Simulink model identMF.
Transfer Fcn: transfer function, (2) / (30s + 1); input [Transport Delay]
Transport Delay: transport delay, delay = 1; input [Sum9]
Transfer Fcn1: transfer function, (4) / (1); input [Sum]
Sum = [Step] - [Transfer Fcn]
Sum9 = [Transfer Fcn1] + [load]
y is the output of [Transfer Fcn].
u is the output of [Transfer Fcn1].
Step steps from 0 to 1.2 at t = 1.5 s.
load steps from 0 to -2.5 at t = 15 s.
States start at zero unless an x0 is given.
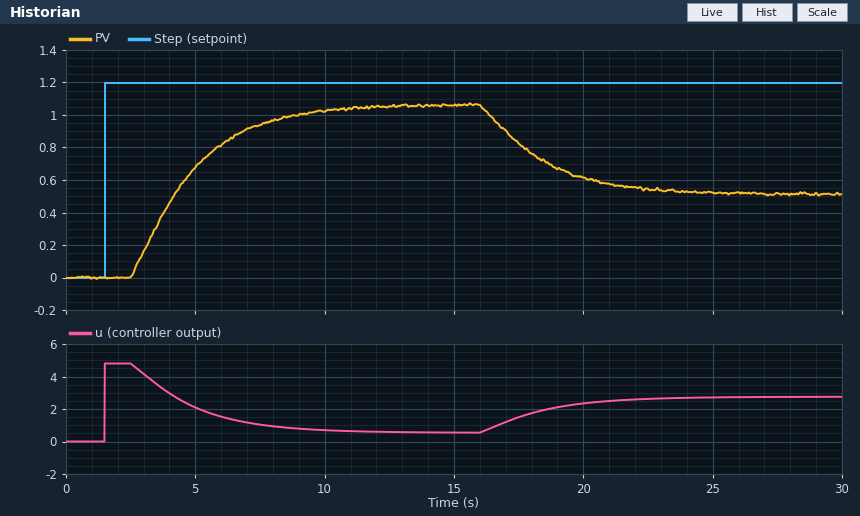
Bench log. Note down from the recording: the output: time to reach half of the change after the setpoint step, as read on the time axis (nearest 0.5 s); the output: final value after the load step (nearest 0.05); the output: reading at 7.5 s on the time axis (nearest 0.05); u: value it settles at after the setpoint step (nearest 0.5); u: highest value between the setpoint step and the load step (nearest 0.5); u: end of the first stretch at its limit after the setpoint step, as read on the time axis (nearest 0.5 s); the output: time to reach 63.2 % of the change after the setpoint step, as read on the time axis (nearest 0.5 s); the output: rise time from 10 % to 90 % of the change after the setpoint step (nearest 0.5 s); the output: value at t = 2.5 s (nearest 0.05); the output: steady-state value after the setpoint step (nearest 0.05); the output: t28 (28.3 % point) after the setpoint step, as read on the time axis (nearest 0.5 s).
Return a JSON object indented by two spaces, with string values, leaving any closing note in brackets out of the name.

{
  "the output: time to reach half of the change after the setpoint step, as read on the time axis": "4.5 s",
  "the output: final value after the load step": "0.50",
  "the output: reading at 7.5 s on the time axis": "0.95",
  "u: value it settles at after the setpoint step": "0.5",
  "u: highest value between the setpoint step and the load step": "5.0",
  "u: end of the first stretch at its limit after the setpoint step, as read on the time axis": "2.5 s",
  "the output: time to reach 63.2 % of the change after the setpoint step, as read on the time axis": "5.0 s",
  "the output: rise time from 10 % to 90 % of the change after the setpoint step": "5.0 s",
  "the output: value at t = 2.5 s": "0.00",
  "the output: steady-state value after the setpoint step": "1.05",
  "the output: t28 (28.3 % point) after the setpoint step, as read on the time axis": "3.5 s"
}
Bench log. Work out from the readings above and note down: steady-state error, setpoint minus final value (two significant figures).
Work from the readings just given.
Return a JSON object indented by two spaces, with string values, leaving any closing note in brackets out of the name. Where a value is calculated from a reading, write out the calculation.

{
  "steady-state error, setpoint minus final value": "1.2 - 1.05 = 0.15"
}
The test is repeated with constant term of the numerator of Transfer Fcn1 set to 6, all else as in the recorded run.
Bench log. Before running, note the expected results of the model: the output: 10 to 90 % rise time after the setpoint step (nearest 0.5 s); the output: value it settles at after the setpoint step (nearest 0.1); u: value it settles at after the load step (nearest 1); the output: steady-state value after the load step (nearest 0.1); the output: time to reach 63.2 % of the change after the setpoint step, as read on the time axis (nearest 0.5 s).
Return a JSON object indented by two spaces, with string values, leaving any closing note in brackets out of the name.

{
  "the output: 10 to 90 % rise time after the setpoint step": "2.5 s",
  "the output: value it settles at after the setpoint step": "1.1",
  "u: value it settles at after the load step": "3",
  "the output: steady-state value after the load step": "0.7",
  "the output: time to reach 63.2 % of the change after the setpoint step, as read on the time axis": "4.0 s"
}
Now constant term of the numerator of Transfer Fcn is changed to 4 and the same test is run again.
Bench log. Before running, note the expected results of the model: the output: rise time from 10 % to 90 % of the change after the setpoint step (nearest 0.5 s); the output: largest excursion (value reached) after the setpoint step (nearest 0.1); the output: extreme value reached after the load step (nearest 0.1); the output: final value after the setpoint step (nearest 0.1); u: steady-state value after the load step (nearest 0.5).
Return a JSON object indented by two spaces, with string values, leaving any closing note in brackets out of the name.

{
  "the output: rise time from 10 % to 90 % of the change after the setpoint step": "1.5 s",
  "the output: largest excursion (value reached) after the setpoint step": "1.2",
  "the output: extreme value reached after the load step": "0.5",
  "the output: final value after the setpoint step": "1.1",
  "u: steady-state value after the load step": "2.5"
}
